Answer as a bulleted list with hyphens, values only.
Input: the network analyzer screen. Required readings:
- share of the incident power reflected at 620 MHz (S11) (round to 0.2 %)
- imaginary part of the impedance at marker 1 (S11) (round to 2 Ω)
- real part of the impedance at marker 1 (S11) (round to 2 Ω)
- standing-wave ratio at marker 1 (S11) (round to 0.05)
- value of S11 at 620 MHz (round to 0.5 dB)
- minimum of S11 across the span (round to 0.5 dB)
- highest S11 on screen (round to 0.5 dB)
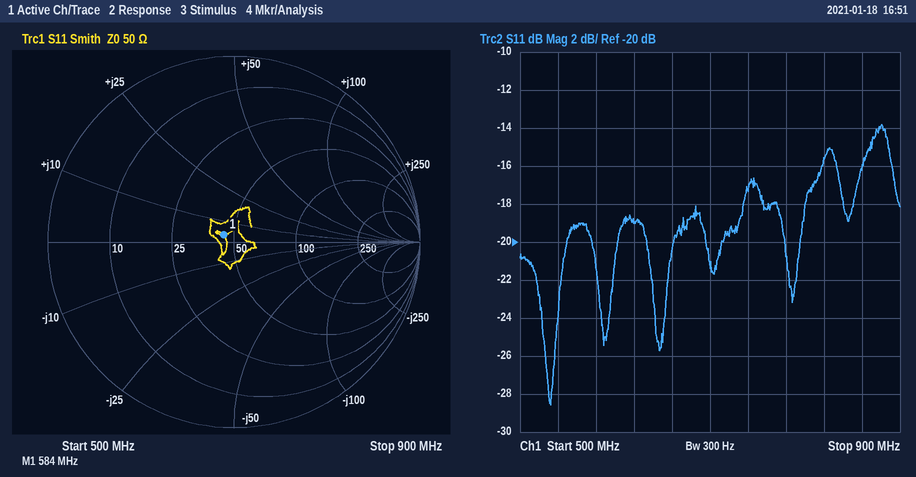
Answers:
- 1.2 %
- +4 Ω
- 44 Ω
- 1.15
- -19.0 dB
- -28.5 dB
- -14.0 dB
